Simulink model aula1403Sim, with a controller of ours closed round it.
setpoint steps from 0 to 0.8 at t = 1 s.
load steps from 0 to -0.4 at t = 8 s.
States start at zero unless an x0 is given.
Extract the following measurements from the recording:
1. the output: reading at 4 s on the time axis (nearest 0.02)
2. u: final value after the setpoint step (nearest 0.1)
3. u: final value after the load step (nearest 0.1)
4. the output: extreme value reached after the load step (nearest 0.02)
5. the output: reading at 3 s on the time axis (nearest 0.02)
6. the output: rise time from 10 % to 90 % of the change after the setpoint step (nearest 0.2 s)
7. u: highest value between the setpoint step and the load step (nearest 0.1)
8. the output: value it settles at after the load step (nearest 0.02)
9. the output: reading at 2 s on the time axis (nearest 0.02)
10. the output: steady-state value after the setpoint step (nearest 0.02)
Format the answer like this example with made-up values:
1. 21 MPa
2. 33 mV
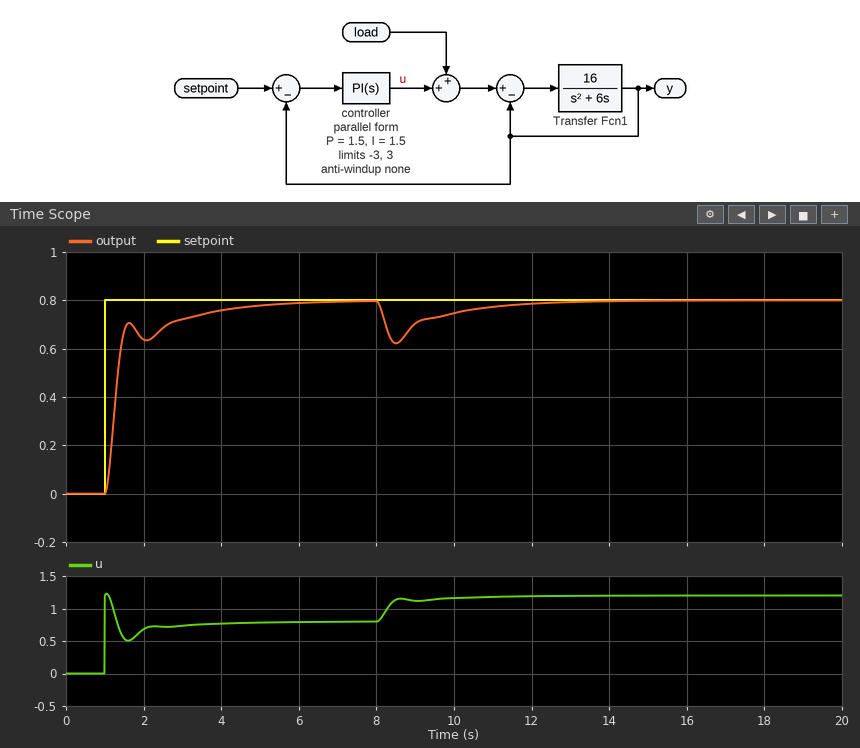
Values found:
1. 0.76
2. 0.8
3. 1.2
4. 0.62
5. 0.72
6. 1.8 s
7. 1.2
8. 0.80
9. 0.64
10. 0.80
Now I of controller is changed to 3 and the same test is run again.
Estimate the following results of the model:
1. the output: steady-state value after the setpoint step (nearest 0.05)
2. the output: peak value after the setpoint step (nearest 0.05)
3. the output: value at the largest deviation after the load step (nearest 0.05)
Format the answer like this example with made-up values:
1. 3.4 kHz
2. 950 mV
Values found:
1. 0.80
2. 0.85
3. 0.65
